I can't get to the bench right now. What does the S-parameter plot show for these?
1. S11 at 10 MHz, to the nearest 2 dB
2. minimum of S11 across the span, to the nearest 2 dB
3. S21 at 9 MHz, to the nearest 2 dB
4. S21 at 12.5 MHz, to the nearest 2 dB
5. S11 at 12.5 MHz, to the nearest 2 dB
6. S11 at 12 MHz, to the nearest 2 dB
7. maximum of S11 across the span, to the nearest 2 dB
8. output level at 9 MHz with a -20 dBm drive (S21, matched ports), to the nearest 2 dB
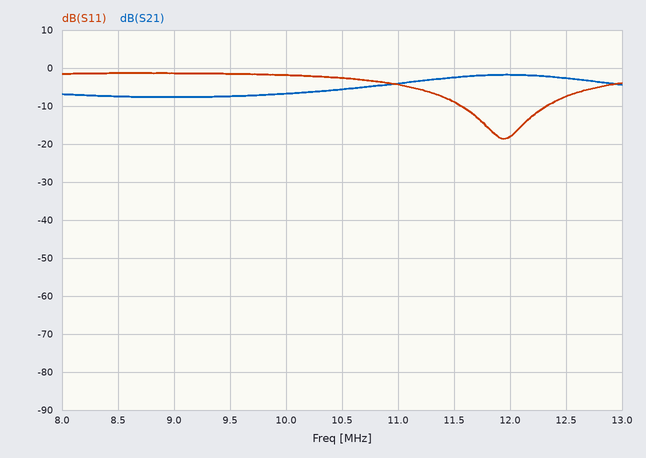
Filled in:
-2 dB
-18 dB
-8 dB
-2 dB
-8 dB
-18 dB
-2 dB
-28 dBm
